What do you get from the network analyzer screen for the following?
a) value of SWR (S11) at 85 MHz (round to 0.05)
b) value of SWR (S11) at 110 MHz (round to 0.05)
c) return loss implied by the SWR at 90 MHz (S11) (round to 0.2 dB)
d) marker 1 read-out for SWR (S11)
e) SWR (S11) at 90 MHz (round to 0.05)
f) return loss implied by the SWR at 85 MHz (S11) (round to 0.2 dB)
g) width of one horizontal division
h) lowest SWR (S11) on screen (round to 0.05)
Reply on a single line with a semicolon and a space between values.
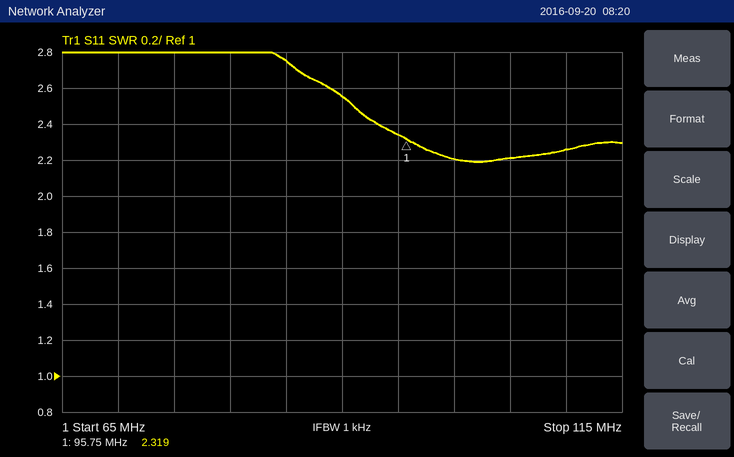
2.75; 2.25; 7.2 dB; 2.319; 2.55; 6.6 dB; 5 MHz; 2.20
